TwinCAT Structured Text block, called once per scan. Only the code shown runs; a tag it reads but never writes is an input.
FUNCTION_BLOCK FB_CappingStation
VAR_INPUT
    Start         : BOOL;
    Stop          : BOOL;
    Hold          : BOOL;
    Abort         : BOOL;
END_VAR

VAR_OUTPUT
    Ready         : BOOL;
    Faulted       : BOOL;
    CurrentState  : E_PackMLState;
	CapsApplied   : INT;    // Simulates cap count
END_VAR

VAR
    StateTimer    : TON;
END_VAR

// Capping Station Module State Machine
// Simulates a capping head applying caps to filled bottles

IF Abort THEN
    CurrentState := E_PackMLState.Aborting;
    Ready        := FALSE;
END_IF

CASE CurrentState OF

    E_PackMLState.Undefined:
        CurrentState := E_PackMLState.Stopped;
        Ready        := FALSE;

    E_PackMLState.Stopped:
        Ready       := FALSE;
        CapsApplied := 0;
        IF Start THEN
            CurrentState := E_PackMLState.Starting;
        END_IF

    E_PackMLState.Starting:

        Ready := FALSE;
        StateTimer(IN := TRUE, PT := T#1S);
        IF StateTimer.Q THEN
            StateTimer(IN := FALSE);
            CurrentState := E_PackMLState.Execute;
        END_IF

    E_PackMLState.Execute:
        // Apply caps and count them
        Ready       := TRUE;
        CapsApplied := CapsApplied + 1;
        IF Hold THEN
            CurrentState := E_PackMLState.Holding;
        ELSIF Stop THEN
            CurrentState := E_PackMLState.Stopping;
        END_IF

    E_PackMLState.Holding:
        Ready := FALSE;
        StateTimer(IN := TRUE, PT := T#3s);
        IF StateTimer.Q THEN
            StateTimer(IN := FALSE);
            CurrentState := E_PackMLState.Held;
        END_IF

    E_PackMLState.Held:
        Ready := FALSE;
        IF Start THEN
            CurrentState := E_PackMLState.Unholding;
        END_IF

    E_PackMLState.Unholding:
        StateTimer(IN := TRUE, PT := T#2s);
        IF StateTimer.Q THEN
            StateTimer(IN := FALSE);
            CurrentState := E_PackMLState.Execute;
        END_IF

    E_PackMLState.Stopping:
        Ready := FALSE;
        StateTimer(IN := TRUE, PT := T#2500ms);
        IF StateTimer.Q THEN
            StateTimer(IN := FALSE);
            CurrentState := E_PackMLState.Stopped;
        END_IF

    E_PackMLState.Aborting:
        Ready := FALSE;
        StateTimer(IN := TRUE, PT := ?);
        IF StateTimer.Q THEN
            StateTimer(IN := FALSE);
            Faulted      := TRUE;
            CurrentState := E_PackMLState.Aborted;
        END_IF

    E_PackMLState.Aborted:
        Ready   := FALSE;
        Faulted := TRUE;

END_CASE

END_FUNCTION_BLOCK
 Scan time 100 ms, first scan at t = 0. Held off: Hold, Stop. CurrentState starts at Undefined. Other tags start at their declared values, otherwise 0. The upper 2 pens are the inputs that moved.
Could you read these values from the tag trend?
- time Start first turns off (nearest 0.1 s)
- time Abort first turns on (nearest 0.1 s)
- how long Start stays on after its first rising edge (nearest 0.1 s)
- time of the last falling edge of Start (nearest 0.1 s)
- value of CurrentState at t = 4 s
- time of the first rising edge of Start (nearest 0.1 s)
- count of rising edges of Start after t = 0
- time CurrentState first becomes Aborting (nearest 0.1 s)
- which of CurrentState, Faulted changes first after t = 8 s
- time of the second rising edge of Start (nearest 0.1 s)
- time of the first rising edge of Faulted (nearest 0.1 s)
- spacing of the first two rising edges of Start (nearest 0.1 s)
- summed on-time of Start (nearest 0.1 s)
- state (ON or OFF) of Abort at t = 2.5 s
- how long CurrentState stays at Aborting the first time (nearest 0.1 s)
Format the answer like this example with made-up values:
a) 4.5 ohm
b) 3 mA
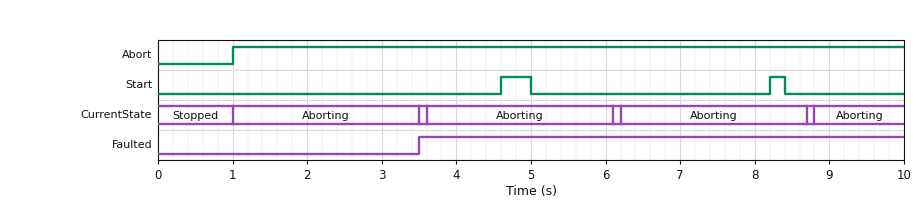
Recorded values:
a) 5.0 s
b) 1.0 s
c) 0.4 s
d) 8.4 s
e) Aborting
f) 4.6 s
g) 2
h) 1.0 s
i) CurrentState
j) 8.2 s
k) 3.5 s
l) 3.6 s
m) 0.6 s
n) ON
o) 2.5 s
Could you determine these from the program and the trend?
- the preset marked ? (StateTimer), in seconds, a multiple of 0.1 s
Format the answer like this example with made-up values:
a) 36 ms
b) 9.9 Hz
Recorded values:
a) 2.5 s
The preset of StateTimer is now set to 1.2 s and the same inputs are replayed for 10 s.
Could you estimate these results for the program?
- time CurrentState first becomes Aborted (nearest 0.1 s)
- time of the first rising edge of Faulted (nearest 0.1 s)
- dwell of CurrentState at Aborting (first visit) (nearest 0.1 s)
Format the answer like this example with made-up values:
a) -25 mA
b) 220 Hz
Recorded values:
a) 2.2 s
b) 2.2 s
c) 1.2 s
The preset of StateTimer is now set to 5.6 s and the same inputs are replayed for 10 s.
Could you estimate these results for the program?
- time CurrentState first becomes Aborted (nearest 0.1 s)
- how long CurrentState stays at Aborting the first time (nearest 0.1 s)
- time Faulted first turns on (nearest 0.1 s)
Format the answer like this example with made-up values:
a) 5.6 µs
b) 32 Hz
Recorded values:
a) 6.6 s
b) 5.6 s
c) 6.6 s
